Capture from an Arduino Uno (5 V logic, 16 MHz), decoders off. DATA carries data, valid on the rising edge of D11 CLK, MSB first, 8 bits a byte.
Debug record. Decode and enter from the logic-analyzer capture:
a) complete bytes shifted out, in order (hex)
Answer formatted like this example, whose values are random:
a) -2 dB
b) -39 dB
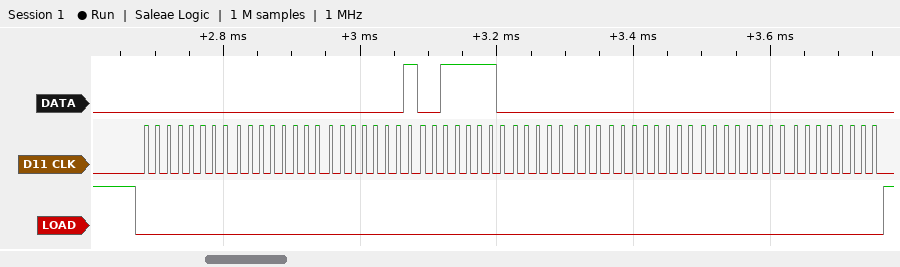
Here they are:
a) 0x00 0x00 0x01 0x3E 0x00 0x00 0x00 0x00
